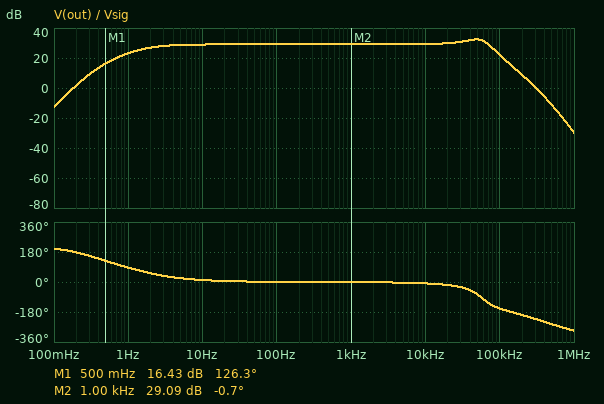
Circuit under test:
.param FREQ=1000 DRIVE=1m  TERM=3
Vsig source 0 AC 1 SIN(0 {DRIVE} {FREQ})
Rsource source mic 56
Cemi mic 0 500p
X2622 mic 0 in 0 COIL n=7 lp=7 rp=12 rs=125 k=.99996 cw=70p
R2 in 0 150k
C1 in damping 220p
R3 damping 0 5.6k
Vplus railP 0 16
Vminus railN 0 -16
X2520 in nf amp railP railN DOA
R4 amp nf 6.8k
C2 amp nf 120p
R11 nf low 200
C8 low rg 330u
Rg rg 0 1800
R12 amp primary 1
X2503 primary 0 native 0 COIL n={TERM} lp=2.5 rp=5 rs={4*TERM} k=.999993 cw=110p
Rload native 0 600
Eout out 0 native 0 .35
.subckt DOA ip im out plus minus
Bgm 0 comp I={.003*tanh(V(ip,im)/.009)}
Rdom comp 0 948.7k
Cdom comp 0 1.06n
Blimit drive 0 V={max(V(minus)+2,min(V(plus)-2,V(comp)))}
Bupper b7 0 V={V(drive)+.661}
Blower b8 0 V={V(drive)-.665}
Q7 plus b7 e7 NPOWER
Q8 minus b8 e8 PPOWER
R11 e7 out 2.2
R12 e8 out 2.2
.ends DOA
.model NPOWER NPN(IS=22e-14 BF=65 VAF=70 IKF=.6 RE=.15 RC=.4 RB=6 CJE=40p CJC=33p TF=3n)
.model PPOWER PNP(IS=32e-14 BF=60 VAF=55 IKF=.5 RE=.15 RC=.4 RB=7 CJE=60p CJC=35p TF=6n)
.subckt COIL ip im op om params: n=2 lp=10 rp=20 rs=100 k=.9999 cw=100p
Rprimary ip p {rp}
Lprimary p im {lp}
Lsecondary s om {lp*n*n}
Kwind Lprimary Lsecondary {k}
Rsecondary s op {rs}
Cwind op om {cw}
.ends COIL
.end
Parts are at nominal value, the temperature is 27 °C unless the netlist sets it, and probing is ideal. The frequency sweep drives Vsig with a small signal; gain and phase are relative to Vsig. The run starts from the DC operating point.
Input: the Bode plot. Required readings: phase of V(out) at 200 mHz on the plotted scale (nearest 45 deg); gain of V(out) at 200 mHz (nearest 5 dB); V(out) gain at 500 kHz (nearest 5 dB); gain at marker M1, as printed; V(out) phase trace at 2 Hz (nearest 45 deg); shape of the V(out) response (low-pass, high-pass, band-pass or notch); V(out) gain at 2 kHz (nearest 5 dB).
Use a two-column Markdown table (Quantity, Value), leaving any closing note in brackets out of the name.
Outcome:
| Quantity | Value |
|---|---|
| phase of V(out) at 200 mHz on the plotted scale | 180 deg |
| gain of V(out) at 200 mHz | 0 dB |
| V(out) gain at 500 kHz | -10 dB |
| gain at marker M1, as printed | 16.43 dB |
| V(out) phase trace at 2 Hz | 45 deg |
| shape of the V(out) response | band-pass |
| V(out) gain at 2 kHz | 30 dB |
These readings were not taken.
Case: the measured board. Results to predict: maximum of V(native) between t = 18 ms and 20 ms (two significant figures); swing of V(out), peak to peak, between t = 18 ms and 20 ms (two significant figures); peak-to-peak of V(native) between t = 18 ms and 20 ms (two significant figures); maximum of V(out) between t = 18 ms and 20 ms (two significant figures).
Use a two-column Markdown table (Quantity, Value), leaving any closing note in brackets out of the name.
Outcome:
| Quantity | Value |
|---|---|
| maximum of V(native) between t = 18 ms and 20 ms | 81 mV |
| swing of V(out), peak to peak, between t = 18 ms and 20 ms | 57 mV |
| peak-to-peak of V(native) between t = 18 ms and 20 ms | 160 mV |
| maximum of V(out) between t = 18 ms and 20 ms | 28 mV |
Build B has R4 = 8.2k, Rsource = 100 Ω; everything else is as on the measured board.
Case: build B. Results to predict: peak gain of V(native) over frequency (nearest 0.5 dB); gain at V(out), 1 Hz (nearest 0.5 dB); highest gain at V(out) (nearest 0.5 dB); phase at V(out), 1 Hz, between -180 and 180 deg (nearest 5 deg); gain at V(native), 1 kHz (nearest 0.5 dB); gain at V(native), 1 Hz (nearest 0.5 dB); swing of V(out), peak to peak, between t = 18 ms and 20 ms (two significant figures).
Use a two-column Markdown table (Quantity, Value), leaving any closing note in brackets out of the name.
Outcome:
| Quantity | Value |
|---|---|
| peak gain of V(native) over frequency | 41.0 dB |
| gain at V(out), 1 Hz | 21.0 dB |
| highest gain at V(out) | 31.5 dB |
| phase at V(out), 1 Hz, between -180 and 180 deg | 100 deg |
| gain at V(native), 1 kHz | 39.5 dB |
| gain at V(native), 1 Hz | 30.0 dB |
| swing of V(out), peak to peak, between t = 18 ms and 20 ms | 65 mV |
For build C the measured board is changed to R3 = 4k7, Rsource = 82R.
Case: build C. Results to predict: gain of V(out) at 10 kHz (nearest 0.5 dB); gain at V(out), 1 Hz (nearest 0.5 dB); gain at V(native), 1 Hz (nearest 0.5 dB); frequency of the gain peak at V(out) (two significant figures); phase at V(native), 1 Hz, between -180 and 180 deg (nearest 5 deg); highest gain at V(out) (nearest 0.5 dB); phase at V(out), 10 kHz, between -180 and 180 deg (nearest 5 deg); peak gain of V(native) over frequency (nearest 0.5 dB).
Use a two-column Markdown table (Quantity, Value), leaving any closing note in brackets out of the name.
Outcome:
| Quantity | Value |
|---|---|
| gain of V(out) at 10 kHz | 29.0 dB |
| gain at V(out), 1 Hz | 21.0 dB |
| gain at V(native), 1 Hz | 30.0 dB |
| frequency of the gain peak at V(out) | 47 kHz |
| phase at V(native), 1 Hz, between -180 and 180 deg | 95 deg |
| highest gain at V(out) | 31.5 dB |
| phase at V(out), 10 kHz, between -180 and 180 deg | -10 deg |
| peak gain of V(native) over frequency | 40.5 dB |
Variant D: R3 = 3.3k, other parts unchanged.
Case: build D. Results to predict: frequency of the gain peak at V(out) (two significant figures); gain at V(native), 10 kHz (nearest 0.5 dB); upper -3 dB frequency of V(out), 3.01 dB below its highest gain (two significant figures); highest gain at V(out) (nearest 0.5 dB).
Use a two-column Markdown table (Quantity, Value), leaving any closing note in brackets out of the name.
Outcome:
| Quantity | Value |
|---|---|
| frequency of the gain peak at V(out) | 51 kHz |
| gain at V(native), 10 kHz | 38.5 dB |
| upper -3 dB frequency of V(out), 3.01 dB below its highest gain | 67 kHz |
| highest gain at V(out) | 33.5 dB |
